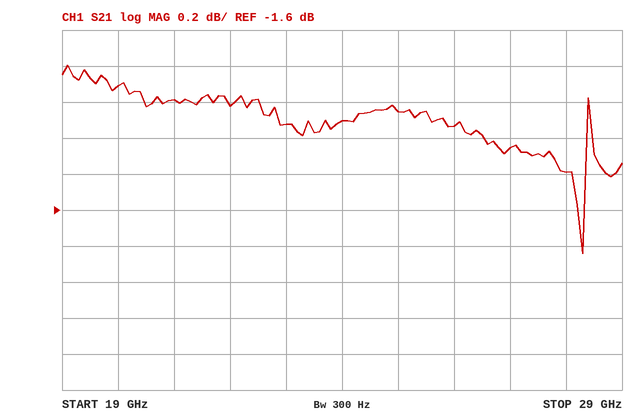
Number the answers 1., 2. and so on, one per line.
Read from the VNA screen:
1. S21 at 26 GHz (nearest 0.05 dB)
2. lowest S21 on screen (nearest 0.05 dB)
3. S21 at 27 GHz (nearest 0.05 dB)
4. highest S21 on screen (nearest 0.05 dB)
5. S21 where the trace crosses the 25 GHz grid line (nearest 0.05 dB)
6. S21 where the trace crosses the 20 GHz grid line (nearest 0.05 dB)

1. -1.15 dB
2. -1.85 dB
3. -1.25 dB
4. -0.80 dB
5. -1.05 dB
6. -0.90 dB
